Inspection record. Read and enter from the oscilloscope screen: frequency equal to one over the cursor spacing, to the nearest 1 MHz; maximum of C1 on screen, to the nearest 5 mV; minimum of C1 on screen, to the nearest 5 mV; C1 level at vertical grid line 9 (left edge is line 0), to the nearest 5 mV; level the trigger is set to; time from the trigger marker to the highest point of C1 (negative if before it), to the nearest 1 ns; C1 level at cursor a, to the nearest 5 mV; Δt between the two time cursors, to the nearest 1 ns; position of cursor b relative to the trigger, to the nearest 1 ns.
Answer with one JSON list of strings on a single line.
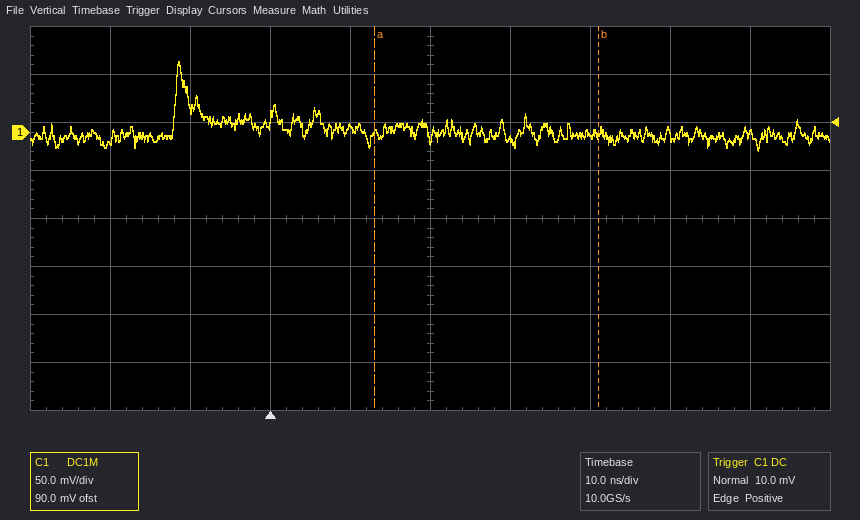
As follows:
["36 MHz", "75 mV", "-20 mV", "0 mV", "10.0 mV", "-11 ns", "0 mV", "28 ns", "+41 ns"]
